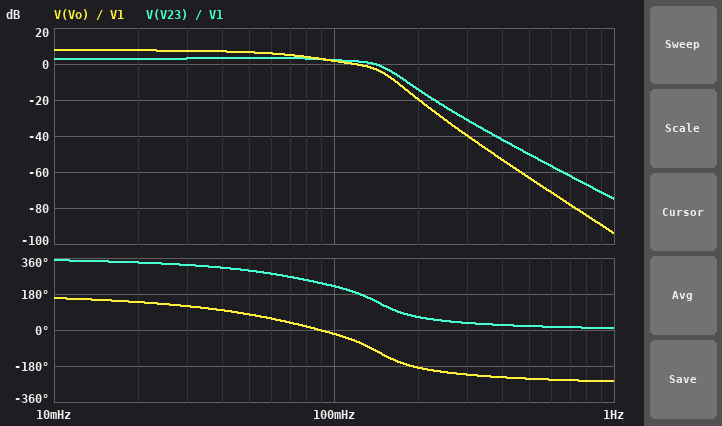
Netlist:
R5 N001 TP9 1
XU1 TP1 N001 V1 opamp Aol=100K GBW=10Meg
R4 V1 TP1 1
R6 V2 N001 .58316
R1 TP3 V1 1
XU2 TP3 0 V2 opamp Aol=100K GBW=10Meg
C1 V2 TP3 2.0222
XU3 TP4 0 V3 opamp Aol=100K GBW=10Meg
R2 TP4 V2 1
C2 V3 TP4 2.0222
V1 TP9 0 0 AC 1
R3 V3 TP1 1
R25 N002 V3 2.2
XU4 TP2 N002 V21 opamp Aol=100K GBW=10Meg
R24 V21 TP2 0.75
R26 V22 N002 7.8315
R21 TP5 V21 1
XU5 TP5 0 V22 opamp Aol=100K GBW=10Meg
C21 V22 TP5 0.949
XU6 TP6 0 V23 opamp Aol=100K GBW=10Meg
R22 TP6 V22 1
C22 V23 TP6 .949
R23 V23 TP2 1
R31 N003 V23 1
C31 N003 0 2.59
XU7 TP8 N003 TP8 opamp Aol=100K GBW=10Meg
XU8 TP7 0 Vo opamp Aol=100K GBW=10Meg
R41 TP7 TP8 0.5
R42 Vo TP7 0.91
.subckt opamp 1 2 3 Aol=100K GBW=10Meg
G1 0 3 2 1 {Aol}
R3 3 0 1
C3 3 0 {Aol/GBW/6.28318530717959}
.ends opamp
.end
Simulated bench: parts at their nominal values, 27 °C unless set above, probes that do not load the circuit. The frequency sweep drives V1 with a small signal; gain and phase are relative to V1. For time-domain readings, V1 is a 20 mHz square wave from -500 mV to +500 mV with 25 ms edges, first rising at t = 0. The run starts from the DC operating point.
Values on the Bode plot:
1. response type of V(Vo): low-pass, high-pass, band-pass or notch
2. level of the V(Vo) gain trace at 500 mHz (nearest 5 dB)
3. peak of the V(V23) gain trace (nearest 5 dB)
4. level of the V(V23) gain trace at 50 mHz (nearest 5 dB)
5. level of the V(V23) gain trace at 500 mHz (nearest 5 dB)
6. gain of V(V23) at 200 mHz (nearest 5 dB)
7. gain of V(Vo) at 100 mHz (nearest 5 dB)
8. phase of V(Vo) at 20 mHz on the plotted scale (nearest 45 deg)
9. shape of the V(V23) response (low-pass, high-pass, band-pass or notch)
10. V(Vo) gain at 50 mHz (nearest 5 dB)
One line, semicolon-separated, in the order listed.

low-pass; -65 dB; 5 dB; 5 dB; -50 dB; -15 dB; 0 dB; 135 deg; low-pass; 5 dB
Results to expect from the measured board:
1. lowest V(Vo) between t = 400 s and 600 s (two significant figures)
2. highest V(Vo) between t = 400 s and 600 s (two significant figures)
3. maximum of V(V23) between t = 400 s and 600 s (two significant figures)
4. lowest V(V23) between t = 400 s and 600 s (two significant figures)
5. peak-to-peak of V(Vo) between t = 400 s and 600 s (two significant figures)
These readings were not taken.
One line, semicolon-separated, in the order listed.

-1.3 V; 1.3 V; 930 mV; -930 mV; 2.5 V
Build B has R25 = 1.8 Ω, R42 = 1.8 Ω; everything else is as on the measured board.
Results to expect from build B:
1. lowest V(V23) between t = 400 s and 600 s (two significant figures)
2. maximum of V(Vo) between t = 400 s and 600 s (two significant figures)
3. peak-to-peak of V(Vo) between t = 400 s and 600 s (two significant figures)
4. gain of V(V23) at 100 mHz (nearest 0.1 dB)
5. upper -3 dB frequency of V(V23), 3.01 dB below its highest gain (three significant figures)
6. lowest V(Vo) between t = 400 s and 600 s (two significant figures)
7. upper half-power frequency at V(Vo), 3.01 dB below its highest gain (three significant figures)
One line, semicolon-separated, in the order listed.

-990 mV; 2.6 V; 5.2 V; 2.8 dB; 145 mHz; -2.6 V; 73.1 mHz
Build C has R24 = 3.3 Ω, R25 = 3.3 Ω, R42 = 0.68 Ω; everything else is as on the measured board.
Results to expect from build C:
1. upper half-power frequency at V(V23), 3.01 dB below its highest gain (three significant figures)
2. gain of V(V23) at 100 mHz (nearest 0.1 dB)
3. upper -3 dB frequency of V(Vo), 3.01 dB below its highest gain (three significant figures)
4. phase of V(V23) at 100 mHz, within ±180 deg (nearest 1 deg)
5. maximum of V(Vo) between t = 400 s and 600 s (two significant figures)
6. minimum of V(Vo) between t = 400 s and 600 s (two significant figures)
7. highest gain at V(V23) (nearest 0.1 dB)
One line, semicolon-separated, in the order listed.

89.3 mHz; -7.4 dB; 59.4 mHz; -125 deg; 470 mV; -470 mV; -3.1 dB
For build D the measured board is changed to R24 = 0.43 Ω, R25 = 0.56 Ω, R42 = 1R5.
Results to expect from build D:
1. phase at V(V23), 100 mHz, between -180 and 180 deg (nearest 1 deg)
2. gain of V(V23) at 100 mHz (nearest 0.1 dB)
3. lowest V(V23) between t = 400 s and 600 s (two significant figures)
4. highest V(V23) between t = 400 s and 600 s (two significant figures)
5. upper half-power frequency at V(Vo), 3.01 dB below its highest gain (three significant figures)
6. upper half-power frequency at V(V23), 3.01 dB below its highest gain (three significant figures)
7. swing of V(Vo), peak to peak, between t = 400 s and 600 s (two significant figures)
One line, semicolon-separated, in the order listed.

-148 deg; 15.7 dB; -2.3 V; 2.3 V; 115 mHz; 116 mHz; 9.1 V
